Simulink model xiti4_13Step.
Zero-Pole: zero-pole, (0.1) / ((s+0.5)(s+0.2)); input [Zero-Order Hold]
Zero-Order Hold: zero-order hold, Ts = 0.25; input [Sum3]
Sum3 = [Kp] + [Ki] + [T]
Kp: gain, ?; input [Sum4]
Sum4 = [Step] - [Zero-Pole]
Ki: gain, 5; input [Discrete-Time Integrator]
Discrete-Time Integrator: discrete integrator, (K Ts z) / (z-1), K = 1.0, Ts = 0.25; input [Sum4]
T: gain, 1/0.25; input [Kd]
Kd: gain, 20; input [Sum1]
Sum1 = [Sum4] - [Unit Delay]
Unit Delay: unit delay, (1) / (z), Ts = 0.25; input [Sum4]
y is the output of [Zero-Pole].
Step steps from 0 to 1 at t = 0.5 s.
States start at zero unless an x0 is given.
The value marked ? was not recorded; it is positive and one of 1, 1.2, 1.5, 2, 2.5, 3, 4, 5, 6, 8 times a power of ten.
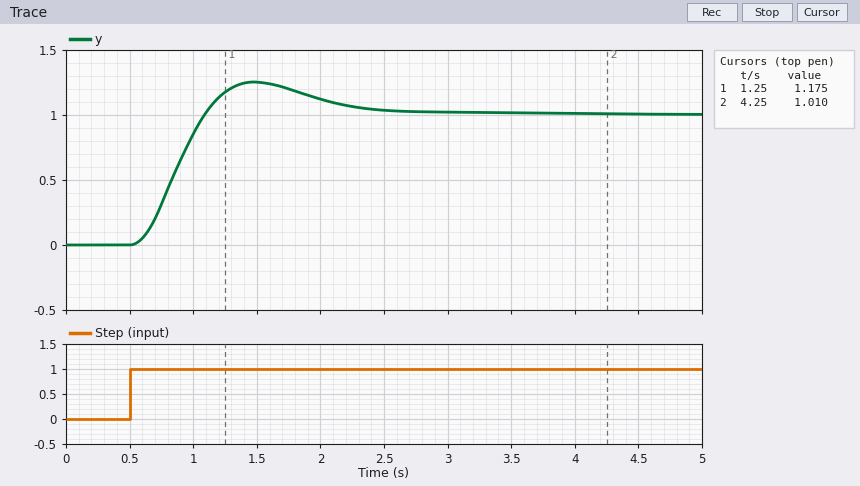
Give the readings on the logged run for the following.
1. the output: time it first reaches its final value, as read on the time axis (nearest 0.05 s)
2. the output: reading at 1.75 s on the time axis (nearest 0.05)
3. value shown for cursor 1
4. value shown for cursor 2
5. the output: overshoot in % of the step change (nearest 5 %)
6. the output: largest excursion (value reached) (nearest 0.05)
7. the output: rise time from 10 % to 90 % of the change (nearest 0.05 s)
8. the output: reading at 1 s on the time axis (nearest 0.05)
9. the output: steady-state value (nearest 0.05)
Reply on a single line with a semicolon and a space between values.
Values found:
1.10 s; 1.20; 1.175; 1.010; 25 %; 1.25; 0.40 s; 0.85; 1.00
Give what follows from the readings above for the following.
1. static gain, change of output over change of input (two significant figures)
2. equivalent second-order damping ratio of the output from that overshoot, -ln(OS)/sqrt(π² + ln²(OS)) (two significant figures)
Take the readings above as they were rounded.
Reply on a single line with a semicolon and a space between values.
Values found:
1.0; 0.40
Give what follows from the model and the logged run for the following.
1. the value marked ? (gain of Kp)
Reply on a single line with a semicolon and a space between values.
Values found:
25
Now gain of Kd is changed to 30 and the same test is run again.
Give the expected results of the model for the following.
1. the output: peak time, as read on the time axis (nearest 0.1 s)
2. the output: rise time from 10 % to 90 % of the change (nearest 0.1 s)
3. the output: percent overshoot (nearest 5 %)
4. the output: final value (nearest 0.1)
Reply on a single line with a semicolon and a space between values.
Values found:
1.2 s; 0.3 s; 30 %; 1.0
